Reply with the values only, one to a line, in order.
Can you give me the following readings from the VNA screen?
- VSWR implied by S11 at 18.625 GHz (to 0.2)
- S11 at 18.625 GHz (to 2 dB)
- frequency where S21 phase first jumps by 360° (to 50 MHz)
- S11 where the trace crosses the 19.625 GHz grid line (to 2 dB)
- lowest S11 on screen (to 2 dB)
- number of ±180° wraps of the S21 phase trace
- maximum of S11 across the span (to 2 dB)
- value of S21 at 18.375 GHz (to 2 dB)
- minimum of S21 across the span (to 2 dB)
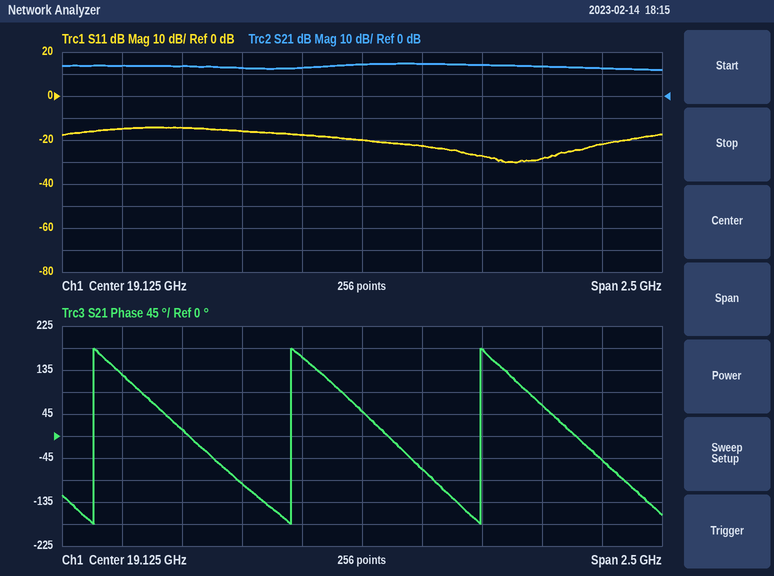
1.4
-16 dB
18.00 GHz
-28 dB
-30 dB
3
-14 dB
14 dB
12 dB
